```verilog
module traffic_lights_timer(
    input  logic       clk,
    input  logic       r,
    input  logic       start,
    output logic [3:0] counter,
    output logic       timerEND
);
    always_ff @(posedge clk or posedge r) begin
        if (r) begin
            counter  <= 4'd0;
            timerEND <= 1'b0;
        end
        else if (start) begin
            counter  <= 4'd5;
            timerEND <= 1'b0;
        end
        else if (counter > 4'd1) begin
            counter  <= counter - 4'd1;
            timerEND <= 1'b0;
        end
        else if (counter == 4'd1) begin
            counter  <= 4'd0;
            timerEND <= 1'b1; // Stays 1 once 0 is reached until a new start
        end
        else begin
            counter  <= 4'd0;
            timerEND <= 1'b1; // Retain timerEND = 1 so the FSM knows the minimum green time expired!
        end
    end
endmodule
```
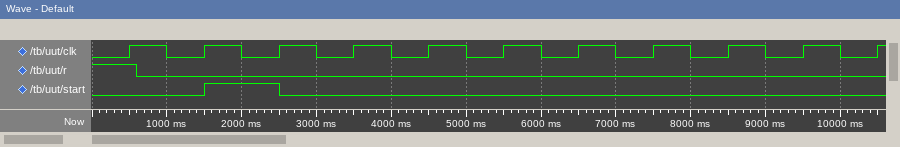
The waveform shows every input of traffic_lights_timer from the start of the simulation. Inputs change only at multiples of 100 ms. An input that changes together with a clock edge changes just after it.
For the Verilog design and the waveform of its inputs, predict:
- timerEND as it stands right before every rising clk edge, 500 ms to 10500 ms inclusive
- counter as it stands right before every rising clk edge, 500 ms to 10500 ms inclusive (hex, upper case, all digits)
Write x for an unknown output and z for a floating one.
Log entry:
0 0 1 0 0 0 0 0 1 1 1
0, 0, 0, 5, 4, 3, 2, 1, 0, 0, 0
